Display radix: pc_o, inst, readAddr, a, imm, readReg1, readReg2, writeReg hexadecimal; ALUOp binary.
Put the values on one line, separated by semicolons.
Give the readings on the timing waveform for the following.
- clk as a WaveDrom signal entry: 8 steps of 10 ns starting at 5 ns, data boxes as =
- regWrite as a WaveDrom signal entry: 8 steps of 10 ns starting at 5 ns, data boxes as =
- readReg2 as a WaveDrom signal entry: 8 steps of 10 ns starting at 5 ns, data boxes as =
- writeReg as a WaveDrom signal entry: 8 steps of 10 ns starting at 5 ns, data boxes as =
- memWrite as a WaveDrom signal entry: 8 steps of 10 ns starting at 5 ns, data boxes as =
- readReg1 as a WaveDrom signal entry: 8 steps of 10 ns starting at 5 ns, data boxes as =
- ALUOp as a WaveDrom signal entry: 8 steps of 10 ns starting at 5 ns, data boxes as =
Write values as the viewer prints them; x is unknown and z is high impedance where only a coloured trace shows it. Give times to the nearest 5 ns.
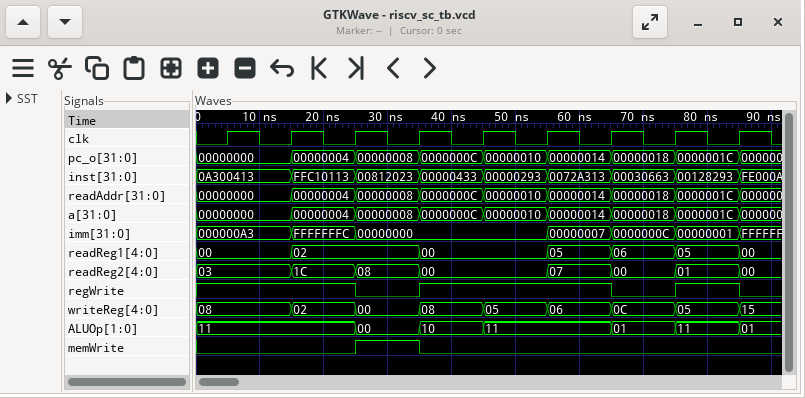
{name: 'clk', wave: 'p.......'}; {name: 'regWrite', wave: '1.01..01'}; {name: 'readReg2', wave: '====.===', data: '03 1C 08 00 07 00 01'}; {name: 'writeReg', wave: '========', data: '08 02 00 08 05 06 0C 05'}; {name: 'memWrite', wave: '0.10....'}; {name: 'readReg1', wave: '==.=.===', data: '00 02 00 05 06 05'}; {name: 'ALUOp', wave: '=.===.==', data: '11 00 10 11 01 11'}
